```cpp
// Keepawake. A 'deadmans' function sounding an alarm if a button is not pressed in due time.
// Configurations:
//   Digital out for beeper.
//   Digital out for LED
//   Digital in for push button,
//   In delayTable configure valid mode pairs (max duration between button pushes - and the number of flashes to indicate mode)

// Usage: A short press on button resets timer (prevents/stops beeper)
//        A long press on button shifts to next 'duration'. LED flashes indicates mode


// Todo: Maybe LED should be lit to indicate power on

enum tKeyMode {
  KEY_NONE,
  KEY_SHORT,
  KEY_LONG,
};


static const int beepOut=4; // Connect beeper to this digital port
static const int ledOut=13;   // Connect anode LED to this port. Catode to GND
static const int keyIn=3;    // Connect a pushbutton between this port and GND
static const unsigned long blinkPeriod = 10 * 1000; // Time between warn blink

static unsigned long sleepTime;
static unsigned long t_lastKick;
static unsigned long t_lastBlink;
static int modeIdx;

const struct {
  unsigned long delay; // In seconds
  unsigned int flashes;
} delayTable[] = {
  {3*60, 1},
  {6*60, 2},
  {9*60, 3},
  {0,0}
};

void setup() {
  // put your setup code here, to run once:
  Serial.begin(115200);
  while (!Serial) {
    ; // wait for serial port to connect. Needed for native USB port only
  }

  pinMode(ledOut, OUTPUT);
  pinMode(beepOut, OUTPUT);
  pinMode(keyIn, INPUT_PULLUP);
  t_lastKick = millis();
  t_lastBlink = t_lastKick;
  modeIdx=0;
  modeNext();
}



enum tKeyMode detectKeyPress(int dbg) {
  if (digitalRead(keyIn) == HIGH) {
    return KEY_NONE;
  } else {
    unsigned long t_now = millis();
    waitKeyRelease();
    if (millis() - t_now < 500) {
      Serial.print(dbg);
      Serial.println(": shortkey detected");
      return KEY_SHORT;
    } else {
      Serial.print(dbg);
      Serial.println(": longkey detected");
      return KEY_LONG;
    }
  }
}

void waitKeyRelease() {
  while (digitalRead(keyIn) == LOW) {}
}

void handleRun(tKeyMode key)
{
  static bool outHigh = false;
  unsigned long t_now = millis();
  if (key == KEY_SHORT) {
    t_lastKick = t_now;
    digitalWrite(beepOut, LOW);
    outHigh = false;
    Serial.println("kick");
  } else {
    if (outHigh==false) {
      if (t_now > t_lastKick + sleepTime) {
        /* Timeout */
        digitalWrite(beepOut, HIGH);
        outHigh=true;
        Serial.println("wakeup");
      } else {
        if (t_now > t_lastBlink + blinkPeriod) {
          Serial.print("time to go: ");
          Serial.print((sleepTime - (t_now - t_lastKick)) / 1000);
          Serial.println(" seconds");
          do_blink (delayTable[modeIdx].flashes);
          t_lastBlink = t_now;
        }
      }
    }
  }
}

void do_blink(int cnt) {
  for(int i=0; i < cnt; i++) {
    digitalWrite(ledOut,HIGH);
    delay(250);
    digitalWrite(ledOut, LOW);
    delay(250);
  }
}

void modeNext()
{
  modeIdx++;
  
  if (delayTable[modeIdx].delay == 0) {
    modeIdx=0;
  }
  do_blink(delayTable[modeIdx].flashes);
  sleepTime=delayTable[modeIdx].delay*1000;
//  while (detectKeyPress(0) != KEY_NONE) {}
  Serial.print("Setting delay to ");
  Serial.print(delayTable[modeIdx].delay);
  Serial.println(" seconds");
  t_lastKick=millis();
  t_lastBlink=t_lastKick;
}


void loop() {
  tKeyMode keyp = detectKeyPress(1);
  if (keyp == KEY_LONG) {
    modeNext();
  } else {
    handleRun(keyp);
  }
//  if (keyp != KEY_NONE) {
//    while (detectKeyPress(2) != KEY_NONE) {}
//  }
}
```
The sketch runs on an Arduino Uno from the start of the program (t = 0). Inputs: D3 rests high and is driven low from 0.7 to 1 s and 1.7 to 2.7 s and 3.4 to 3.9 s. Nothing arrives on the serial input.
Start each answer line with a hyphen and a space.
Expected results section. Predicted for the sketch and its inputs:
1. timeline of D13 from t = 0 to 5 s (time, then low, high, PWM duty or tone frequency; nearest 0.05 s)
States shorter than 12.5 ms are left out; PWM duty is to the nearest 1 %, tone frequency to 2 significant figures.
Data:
- 0 s high; 0.25 s low; 0.5 s high; 0.75 s low; 2.7 s high; 2.95 s low; 3.2 s high; 3.45 s low; 3.7 s high; 3.95 s low
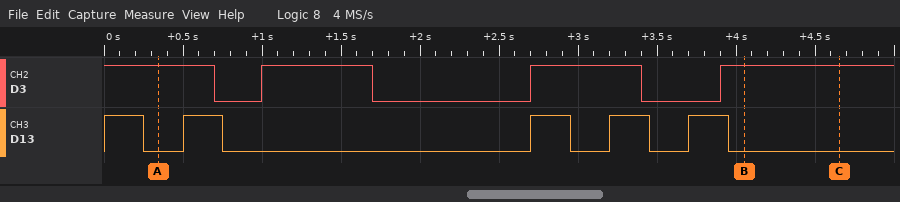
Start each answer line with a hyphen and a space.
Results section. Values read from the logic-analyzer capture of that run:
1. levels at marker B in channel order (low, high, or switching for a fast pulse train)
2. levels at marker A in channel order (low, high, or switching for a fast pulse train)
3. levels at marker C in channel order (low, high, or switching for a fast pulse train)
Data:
- D3 high, D13 low
- D3 high, D13 low
- D3 high, D13 low
